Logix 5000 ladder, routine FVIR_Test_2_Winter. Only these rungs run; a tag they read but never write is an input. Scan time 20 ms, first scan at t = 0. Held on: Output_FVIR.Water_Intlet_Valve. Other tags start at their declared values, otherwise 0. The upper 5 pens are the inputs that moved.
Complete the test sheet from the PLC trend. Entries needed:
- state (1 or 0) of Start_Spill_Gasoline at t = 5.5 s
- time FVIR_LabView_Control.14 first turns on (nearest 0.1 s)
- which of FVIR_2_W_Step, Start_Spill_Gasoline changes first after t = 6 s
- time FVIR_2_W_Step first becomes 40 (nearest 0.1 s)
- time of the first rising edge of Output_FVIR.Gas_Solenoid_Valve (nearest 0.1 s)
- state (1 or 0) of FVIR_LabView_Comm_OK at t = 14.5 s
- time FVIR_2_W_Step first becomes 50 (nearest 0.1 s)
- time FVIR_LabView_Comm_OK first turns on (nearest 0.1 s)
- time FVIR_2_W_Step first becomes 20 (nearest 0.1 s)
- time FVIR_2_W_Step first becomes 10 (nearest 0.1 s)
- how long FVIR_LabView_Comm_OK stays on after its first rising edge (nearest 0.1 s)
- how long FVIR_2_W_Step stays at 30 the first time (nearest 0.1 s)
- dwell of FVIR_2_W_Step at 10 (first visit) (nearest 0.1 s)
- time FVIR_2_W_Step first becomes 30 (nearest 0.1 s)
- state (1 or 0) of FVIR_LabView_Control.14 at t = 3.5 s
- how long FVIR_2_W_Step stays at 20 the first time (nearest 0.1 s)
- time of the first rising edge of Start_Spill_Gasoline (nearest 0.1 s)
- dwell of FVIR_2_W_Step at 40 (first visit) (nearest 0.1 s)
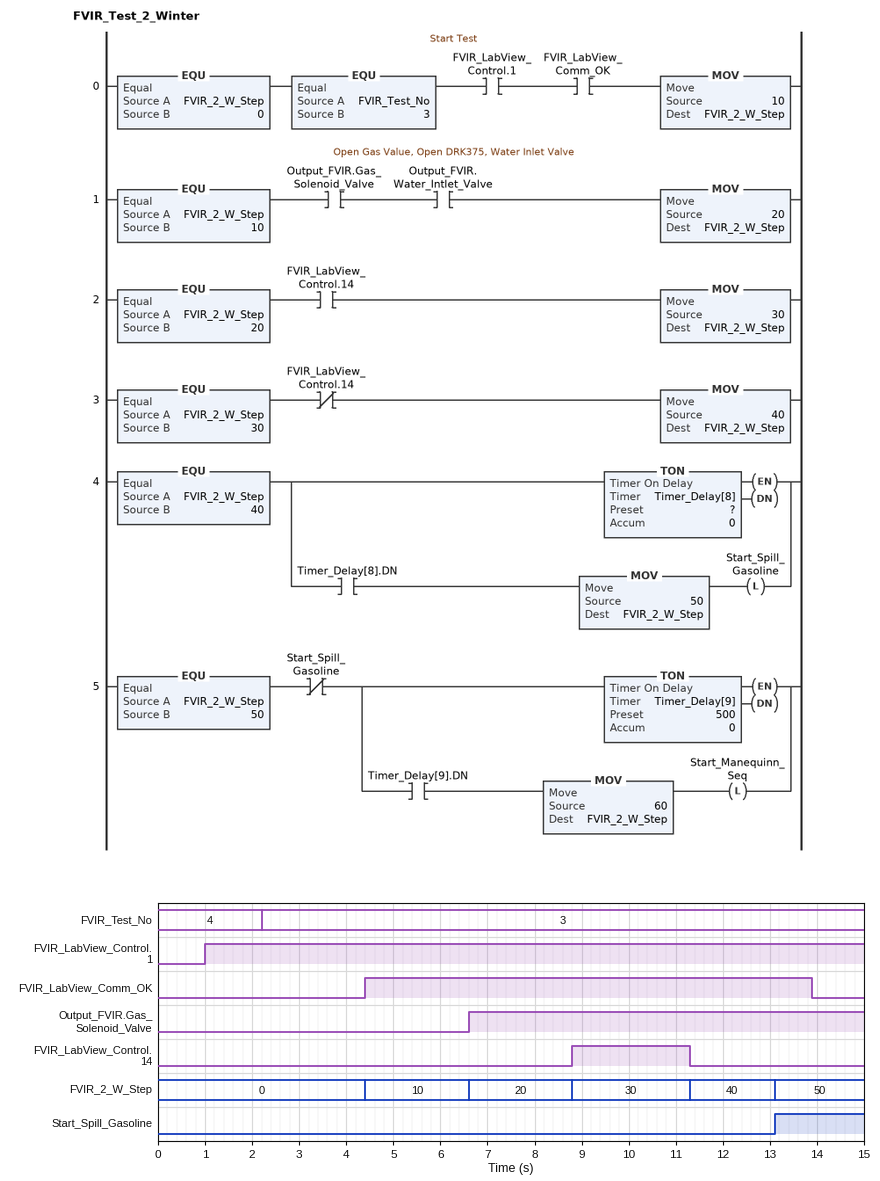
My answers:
0
8.8 s
FVIR_2_W_Step
11.3 s
6.6 s
0
13.1 s
4.4 s
6.6 s
4.4 s
9.5 s
2.5 s
2.2 s
8.8 s
0
2.2 s
13.1 s
1.8 s
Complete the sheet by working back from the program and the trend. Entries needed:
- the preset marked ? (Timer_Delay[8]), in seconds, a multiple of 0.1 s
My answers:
1.8 s
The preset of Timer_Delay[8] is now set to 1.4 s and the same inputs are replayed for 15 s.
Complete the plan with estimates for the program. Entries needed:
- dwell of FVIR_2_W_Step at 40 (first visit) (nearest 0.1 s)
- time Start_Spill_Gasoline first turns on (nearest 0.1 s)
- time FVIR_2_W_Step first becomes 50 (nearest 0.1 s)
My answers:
1.4 s
12.7 s
12.7 s
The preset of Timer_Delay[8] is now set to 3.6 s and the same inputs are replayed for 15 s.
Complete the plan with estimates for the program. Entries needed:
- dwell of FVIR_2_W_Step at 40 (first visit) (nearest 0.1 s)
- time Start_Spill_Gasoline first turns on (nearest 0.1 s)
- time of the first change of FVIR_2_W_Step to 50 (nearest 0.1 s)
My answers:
3.6 s
14.9 s
14.9 s
